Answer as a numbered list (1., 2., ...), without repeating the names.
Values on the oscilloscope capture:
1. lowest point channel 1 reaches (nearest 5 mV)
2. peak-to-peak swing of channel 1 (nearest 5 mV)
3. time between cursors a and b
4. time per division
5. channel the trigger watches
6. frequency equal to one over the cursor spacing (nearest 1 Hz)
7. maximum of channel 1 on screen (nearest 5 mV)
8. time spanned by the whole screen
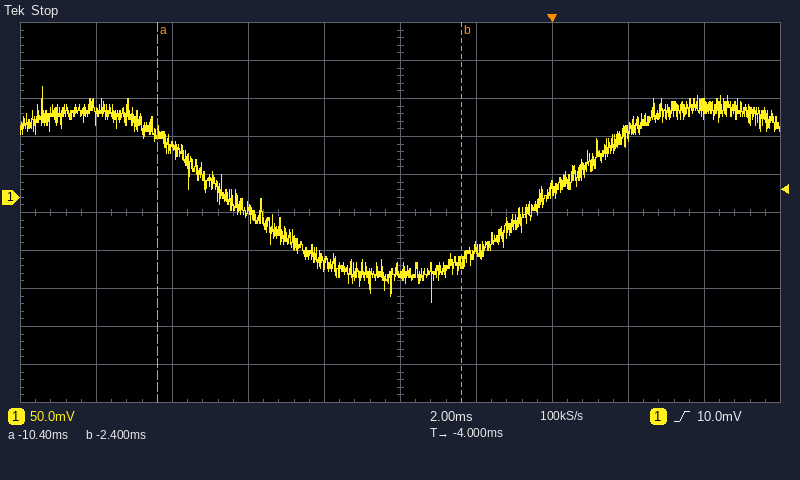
1. -140 mV
2. 285 mV
3. 8.0 ms
4. 2 ms
5. channel 1
6. 125 Hz
7. 145 mV
8. 20 ms
